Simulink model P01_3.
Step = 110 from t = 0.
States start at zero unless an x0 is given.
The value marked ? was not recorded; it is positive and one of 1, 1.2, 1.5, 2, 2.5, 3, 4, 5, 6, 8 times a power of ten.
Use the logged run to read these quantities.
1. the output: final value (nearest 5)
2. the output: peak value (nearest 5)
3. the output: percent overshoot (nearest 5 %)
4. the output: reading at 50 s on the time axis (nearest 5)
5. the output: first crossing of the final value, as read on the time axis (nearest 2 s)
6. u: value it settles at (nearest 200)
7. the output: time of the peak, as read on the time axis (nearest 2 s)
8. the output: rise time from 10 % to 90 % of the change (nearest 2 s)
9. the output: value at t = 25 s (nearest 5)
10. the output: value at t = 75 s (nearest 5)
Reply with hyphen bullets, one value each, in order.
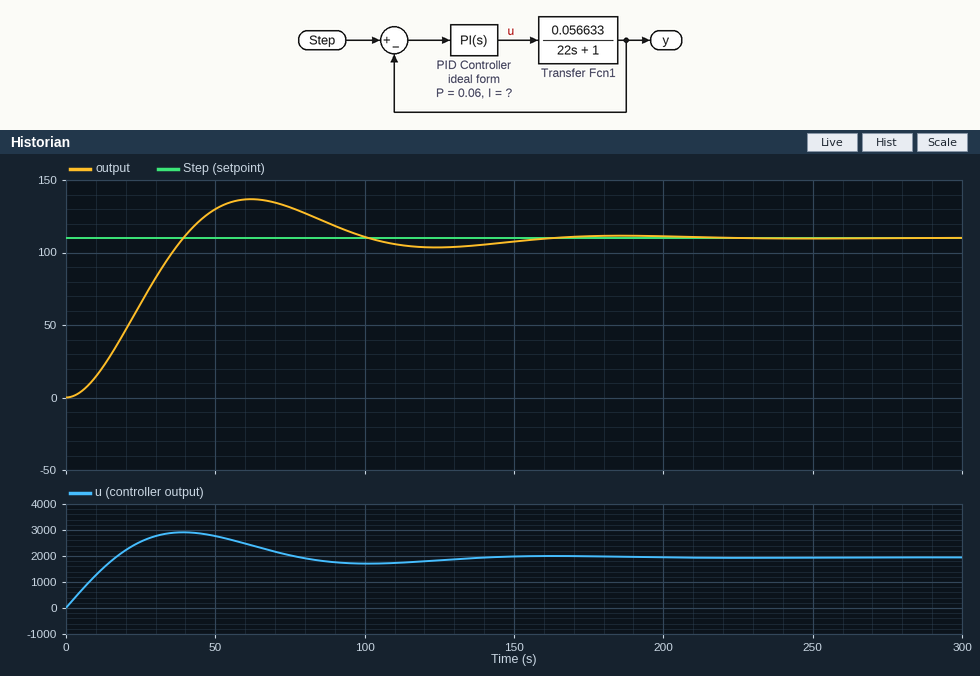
- 110
- 135
- 25 %
- 130
- 40 s
- 2000
- 62 s
- 26 s
- 65
- 130
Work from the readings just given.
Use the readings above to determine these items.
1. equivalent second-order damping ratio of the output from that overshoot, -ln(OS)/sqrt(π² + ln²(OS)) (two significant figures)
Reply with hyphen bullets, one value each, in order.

- 0.40
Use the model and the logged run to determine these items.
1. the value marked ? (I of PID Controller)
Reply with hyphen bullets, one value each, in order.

- 20
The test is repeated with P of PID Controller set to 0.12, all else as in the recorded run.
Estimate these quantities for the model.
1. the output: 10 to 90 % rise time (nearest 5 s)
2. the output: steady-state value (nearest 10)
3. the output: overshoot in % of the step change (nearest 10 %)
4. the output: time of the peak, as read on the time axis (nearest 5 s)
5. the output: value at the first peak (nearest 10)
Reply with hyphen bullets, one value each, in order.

- 15 s
- 110
- 40 %
- 40 s
- 150
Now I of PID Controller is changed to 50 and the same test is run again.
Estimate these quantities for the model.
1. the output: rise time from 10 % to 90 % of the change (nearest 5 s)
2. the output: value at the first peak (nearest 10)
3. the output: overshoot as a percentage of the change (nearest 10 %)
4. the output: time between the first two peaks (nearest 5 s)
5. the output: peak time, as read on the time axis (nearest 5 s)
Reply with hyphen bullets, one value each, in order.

- 15 s
- 160
- 40 %
- 75 s
- 35 s
